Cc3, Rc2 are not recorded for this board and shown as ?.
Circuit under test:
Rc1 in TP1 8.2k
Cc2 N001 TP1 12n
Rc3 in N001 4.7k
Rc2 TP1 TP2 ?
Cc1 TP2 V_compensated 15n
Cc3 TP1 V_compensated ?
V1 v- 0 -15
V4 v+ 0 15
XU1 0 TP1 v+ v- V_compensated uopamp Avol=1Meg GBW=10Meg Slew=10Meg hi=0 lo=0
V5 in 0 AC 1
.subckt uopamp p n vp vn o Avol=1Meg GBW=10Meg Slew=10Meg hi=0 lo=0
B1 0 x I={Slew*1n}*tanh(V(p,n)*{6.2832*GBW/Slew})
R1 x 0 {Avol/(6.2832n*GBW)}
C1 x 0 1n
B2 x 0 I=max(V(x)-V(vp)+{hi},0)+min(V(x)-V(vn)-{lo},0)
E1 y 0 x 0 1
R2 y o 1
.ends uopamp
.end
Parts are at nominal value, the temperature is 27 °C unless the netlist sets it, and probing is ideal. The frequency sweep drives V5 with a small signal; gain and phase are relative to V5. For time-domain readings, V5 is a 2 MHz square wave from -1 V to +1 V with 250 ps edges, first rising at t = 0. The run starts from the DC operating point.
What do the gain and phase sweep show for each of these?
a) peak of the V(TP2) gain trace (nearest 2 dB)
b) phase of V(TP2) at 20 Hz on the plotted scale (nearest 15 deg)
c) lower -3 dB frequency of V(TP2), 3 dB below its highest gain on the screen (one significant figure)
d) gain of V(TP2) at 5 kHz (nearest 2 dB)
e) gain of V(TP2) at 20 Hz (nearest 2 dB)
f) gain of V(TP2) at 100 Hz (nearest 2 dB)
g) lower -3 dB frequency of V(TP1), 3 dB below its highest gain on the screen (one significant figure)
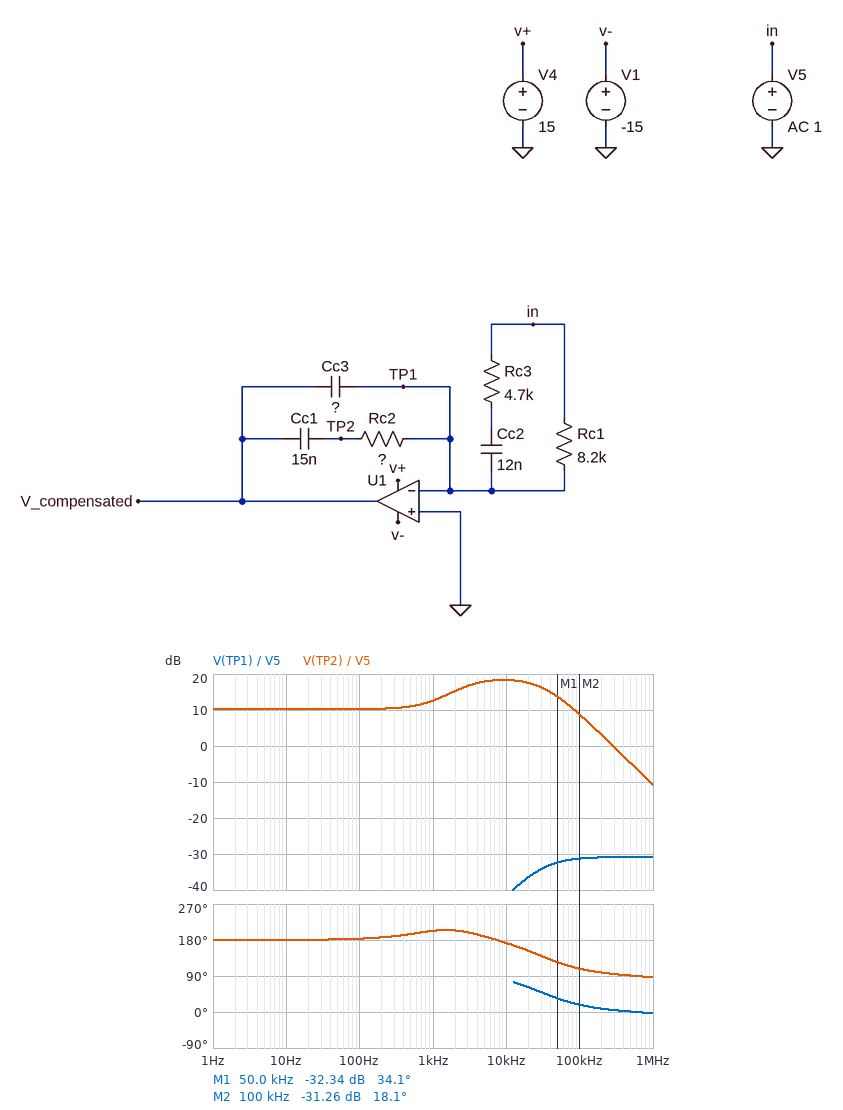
18 dB
180 deg
2 kHz
18 dB
10 dB
10 dB
30 kHz
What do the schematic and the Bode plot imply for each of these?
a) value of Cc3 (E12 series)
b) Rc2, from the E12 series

180 pF
27 kΩ
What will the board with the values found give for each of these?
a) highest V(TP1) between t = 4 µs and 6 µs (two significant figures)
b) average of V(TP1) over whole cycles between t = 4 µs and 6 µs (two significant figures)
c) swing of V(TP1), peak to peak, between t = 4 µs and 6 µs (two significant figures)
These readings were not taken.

25 mV
-110 mV
340 mV
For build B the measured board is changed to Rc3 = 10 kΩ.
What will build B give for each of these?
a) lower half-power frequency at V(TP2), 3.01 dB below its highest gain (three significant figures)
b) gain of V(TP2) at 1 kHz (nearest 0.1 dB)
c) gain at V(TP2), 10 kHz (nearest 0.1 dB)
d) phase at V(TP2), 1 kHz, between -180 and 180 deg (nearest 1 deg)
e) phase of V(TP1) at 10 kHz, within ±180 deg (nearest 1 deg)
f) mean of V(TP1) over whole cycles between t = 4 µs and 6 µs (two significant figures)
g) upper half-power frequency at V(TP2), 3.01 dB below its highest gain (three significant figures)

742 Hz
12.9 dB
15.0 dB
-165 deg
74 deg
-150 mV
34.6 kHz
